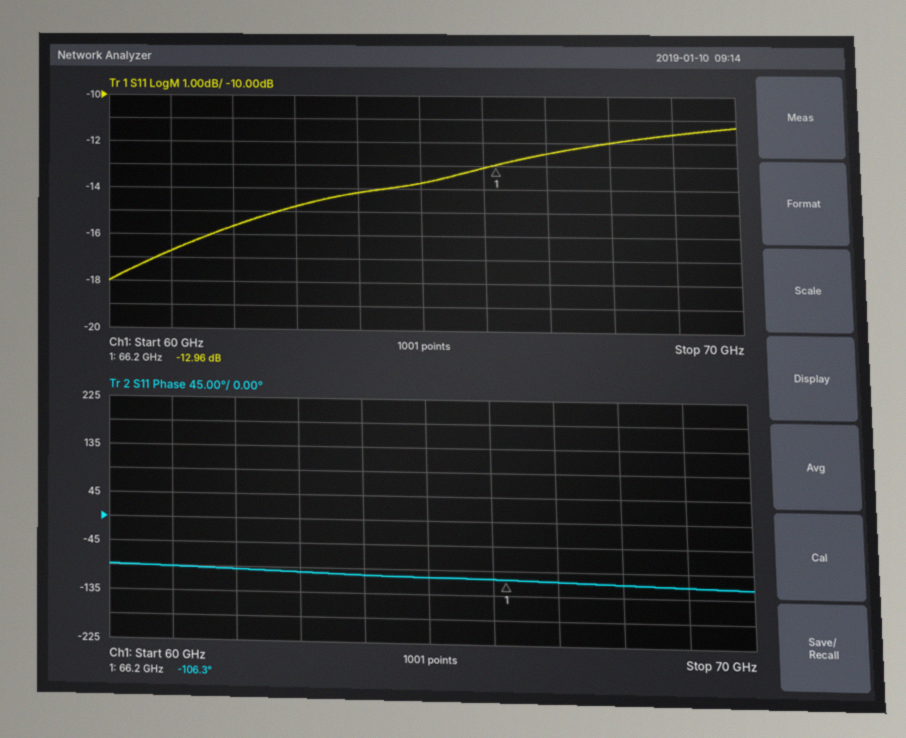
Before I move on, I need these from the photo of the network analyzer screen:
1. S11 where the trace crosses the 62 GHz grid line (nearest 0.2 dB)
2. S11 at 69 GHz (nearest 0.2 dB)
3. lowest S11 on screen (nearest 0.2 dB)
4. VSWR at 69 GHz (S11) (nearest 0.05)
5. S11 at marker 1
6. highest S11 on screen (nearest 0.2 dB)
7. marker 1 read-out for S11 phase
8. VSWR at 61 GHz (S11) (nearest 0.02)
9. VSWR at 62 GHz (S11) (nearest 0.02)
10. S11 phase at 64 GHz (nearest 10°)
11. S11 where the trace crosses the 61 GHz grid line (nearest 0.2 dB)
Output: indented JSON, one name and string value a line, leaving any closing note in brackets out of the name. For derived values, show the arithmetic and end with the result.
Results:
{
  "S11 where the trace crosses the 62 GHz grid line": "-15.6 dB",
  "S11 at 69 GHz": "-11.6 dB",
  "lowest S11 on screen": "-18.0 dB",
  "VSWR at 69 GHz (S11)": "|Γ| = 10^(-11.6/20) = 0.2630; VSWR = (1 + 0.2630)/(1 − 0.2630) ≈ 1.71, so 1.70 to the nearest 0.05",
  "S11 at marker 1": "-12.96 dB",
  "highest S11 on screen": "-11.4 dB",
  "marker 1 read-out for S11 phase": "-106.3°",
  "VSWR at 61 GHz (S11)": "|Γ| = 10^(-16.8/20) = 0.1445; VSWR = (1 + 0.1445)/(1 − 0.1445) ≈ 1.34",
  "VSWR at 62 GHz (S11)": "|Γ| = 10^(-15.6/20) = 0.1660; VSWR = (1 + 0.1660)/(1 − 0.1660) ≈ 1.40",
  "S11 phase at 64 GHz": "-100°",
  "S11 where the trace crosses the 61 GHz grid line": "-16.8 dB"
}
